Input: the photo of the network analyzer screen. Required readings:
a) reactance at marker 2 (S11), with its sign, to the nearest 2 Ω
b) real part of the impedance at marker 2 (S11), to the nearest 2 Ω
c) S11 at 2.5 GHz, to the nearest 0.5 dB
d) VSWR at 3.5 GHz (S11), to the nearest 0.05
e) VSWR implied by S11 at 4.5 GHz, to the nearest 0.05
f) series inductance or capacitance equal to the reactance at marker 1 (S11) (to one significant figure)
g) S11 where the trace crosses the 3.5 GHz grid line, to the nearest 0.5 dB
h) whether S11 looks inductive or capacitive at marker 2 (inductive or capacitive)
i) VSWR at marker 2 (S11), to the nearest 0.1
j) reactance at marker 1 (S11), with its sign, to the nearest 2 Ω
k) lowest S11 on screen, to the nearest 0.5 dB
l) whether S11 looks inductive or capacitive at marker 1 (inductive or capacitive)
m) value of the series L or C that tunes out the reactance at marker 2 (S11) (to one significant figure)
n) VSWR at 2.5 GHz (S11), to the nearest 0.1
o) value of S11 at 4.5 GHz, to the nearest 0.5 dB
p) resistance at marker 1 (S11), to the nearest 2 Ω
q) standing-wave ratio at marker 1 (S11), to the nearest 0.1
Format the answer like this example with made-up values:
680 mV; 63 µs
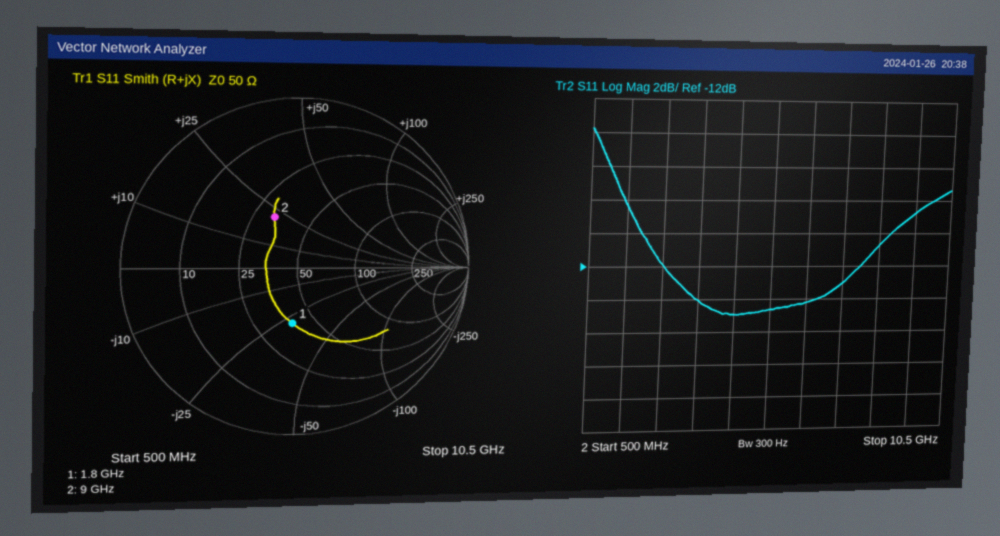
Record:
+22 Ω; 32 Ω; -12.0 dB; 1.50; 1.45; 3 pF; -14.0 dB; inductive; 2.0; -28 Ω; -15.0 dB; capacitive; 800 fF; 1.7; -15.0 dB; 38 Ω; 2.0
